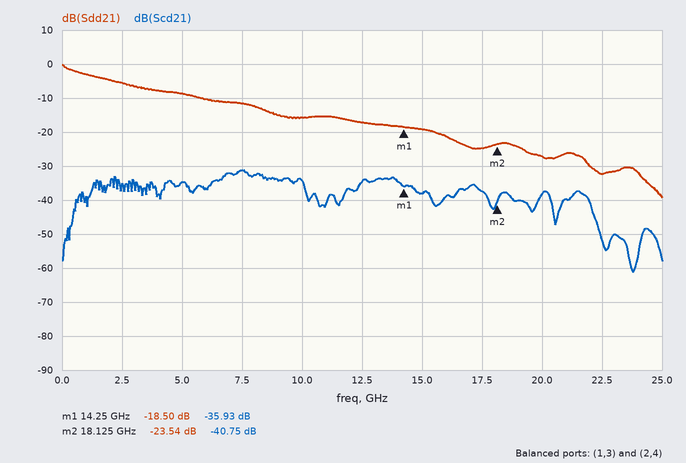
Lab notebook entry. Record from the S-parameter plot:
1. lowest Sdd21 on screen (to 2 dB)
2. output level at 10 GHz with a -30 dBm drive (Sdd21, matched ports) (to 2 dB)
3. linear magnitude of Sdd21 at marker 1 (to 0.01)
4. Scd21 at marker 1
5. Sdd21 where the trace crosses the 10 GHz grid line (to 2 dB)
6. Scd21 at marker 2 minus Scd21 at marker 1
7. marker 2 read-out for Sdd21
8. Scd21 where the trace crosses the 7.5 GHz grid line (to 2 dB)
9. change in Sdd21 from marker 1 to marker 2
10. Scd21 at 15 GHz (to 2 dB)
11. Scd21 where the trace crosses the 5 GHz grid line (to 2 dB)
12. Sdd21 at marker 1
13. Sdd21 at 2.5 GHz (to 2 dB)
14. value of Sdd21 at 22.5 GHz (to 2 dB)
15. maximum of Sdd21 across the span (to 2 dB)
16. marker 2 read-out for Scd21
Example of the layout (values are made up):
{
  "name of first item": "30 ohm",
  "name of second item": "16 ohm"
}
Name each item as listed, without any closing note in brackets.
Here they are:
{
  "lowest Sdd21 on screen": "-40 dB",
  "output level at 10 GHz with a -30 dBm drive (Sdd21, matched ports)": "-46 dBm",
  "linear magnitude of Sdd21 at marker 1": "0.12",
  "Scd21 at marker 1": "-35.93 dB",
  "Sdd21 where the trace crosses the 10 GHz grid line": "-16 dB",
  "Scd21 at marker 2 minus Scd21 at marker 1": "-4.82 dB",
  "marker 2 read-out for Sdd21": "-23.54 dB",
  "Scd21 where the trace crosses the 7.5 GHz grid line": "-32 dB",
  "change in Sdd21 from marker 1 to marker 2": "-5.04 dB",
  "Scd21 at 15 GHz": "-38 dB",
  "Scd21 where the trace crosses the 5 GHz grid line": "-34 dB",
  "Sdd21 at marker 1": "-18.50 dB",
  "Sdd21 at 2.5 GHz": "-6 dB",
  "value of Sdd21 at 22.5 GHz": "-32 dB",
  "maximum of Sdd21 across the span": "0 dB",
  "marker 2 read-out for Scd21": "-40.75 dB"
}
